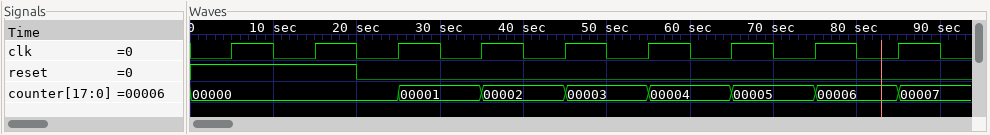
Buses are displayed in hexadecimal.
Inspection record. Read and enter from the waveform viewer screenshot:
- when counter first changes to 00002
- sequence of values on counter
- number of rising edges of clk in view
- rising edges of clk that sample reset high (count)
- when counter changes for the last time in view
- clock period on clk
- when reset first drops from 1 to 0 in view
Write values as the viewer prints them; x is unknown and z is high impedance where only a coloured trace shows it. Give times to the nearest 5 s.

35 s
00000, 00001, 00002, 00003, 00004, 00005, 00006, 00007
9
2
85 s
10 s
20 s
